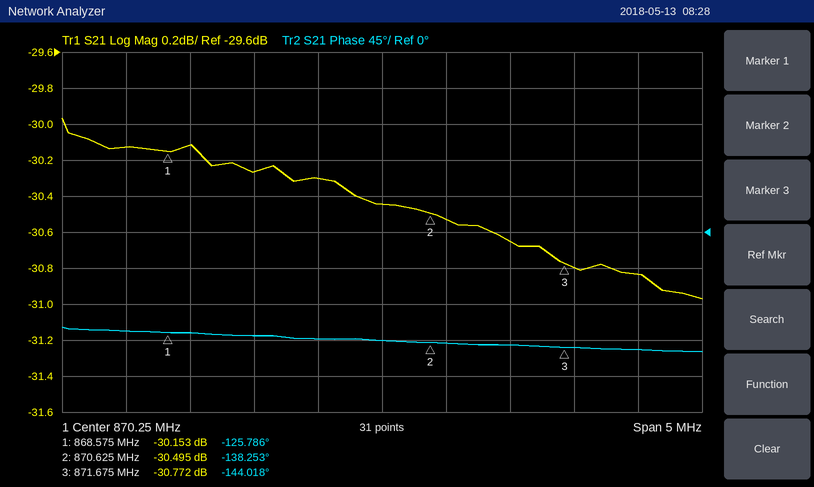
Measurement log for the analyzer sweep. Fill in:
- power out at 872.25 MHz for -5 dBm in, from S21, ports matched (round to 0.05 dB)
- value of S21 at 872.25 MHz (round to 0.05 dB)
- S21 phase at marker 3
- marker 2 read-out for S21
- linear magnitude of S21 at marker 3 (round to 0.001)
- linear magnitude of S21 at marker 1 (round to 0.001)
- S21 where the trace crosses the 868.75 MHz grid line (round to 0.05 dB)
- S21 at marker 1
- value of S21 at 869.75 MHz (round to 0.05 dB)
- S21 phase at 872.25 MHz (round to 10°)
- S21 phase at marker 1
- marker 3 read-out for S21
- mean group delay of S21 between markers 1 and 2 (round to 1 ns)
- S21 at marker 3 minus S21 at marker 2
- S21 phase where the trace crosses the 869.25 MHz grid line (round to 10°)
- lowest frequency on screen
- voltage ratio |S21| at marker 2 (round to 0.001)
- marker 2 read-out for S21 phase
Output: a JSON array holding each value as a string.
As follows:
["-35.85 dBm", "-30.85 dB", "-144.018°", "-30.495 dB", "0.029", "0.031", "-30.10 dB", "-30.153 dB", "-30.30 dB", "-150°", "-125.786°", "-30.772 dB", "17 ns", "-0.277 dB", "-130°", "867.75 MHz", "0.030", "-138.253°"]
